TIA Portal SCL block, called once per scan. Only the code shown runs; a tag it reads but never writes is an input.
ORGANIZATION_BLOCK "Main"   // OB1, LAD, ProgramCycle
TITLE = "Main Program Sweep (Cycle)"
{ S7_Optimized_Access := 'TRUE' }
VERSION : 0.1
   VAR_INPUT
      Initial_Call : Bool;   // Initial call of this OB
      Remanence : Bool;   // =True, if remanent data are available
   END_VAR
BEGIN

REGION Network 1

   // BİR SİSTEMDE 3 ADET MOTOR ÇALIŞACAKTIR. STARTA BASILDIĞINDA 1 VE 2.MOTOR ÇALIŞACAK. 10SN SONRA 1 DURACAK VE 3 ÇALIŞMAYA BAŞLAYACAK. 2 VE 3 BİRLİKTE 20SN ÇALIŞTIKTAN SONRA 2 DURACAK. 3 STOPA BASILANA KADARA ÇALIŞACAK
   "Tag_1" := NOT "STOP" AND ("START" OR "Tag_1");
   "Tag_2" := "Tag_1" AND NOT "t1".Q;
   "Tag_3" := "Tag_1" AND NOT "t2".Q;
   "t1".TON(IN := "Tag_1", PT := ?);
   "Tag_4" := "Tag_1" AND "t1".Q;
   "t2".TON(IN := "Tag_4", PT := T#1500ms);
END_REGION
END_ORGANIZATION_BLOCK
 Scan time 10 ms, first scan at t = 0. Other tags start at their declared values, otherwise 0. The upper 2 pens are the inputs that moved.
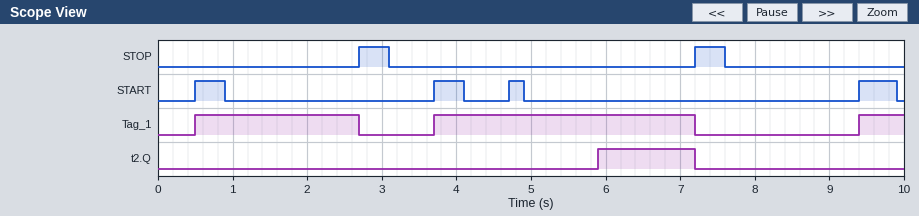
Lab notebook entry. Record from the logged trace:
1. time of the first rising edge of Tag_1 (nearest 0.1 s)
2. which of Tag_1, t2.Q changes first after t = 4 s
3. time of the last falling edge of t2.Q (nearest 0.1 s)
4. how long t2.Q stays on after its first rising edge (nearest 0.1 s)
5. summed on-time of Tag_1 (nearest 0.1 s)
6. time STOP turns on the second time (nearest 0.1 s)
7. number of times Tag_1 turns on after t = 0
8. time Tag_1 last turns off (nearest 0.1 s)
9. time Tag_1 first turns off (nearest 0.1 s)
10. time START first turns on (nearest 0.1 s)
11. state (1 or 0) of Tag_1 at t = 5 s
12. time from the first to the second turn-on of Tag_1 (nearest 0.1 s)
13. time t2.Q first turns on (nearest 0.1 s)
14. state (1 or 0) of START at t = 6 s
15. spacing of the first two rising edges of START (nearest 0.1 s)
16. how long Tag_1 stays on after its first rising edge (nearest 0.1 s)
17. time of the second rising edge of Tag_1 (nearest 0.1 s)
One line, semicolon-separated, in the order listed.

0.5 s; t2.Q; 7.2 s; 1.3 s; 6.3 s; 7.2 s; 3; 7.2 s; 2.7 s; 0.5 s; 1; 3.2 s; 5.9 s; 0; 3.2 s; 2.2 s; 3.7 s
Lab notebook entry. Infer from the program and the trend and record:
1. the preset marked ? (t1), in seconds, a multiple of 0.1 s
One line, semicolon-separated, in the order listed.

0.7 s
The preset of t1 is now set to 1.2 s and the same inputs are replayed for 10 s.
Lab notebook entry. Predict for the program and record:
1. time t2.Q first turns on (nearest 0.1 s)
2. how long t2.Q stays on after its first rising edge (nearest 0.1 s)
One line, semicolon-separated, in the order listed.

6.4 s; 0.8 s
